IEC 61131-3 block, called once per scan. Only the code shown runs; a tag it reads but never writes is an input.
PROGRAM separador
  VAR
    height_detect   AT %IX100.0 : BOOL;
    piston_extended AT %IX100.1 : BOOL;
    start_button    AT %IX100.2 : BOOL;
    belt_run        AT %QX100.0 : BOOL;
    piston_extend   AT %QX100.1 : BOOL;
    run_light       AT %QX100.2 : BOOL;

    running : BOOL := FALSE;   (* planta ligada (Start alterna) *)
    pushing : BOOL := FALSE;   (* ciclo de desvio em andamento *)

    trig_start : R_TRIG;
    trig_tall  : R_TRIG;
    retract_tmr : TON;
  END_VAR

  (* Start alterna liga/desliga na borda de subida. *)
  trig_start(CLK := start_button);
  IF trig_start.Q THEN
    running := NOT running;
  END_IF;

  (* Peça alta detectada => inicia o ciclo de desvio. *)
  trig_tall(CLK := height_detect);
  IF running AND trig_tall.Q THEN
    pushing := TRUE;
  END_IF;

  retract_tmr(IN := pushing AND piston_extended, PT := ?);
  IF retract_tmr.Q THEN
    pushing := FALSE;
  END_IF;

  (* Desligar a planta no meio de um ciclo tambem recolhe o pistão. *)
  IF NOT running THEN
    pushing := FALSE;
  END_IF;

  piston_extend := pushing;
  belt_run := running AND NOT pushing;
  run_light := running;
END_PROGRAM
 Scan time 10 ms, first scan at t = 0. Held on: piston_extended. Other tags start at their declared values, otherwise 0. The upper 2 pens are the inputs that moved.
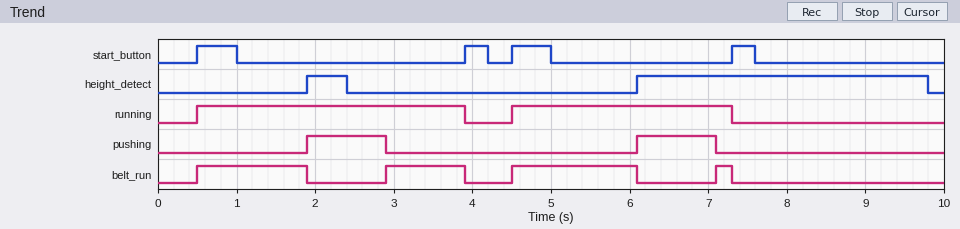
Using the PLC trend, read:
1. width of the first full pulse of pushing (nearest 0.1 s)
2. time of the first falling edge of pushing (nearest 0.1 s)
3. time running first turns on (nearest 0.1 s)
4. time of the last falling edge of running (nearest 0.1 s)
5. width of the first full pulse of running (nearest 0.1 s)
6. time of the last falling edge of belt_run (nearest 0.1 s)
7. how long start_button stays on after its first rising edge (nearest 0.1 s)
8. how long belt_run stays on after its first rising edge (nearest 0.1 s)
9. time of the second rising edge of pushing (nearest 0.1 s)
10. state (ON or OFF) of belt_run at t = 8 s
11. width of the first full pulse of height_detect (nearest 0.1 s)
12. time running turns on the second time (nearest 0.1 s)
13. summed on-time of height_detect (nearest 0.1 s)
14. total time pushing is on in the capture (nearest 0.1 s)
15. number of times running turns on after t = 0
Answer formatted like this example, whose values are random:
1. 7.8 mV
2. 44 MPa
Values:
1. 1.0 s
2. 2.9 s
3. 0.5 s
4. 7.3 s
5. 3.4 s
6. 7.3 s
7. 0.5 s
8. 1.4 s
9. 6.1 s
10. OFF
11. 0.5 s
12. 4.5 s
13. 4.2 s
14. 2.0 s
15. 2
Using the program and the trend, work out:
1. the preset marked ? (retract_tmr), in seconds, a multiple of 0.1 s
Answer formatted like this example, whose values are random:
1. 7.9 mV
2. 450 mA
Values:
1. 1.0 s
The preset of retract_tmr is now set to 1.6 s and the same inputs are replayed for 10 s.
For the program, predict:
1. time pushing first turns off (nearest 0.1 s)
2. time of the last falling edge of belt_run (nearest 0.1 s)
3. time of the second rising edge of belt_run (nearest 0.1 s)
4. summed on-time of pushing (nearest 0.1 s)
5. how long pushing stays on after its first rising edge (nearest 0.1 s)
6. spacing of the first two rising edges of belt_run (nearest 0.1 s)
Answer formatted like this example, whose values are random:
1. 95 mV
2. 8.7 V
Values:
1. 3.5 s
2. 6.1 s
3. 3.5 s
4. 2.8 s
5. 1.6 s
6. 3.0 s
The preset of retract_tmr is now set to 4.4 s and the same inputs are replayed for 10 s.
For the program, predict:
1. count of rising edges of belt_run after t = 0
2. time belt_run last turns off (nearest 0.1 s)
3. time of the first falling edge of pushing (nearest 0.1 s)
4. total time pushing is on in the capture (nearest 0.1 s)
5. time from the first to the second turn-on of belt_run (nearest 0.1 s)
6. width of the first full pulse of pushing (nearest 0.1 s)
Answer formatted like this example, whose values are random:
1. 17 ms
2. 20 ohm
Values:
1. 2
2. 6.1 s
3. 3.9 s
4. 3.2 s
5. 4.0 s
6. 2.0 s
